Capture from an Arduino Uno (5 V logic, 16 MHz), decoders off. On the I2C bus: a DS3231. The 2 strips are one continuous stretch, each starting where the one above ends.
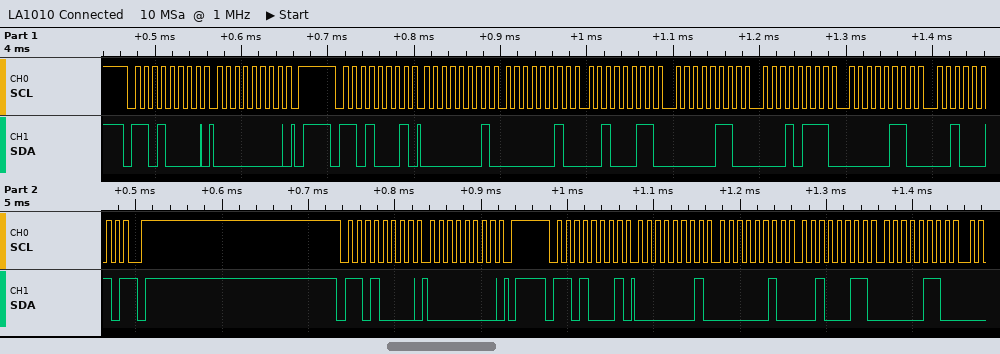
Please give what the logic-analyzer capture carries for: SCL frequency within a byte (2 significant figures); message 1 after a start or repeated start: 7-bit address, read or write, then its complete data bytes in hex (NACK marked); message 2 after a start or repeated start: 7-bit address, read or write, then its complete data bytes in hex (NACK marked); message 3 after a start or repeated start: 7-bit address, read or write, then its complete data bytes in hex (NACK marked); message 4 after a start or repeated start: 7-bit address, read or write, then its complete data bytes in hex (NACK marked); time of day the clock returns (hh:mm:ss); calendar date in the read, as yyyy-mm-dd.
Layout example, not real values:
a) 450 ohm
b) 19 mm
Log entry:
a) 100 kHz
b) 0x68 write: 00
c) 0x68 read: 01 02 23 06 17 06 22 NACK
d) 0x68 write: 00
e) 0x68 read: 01 02 23 06
f) 23:02:01
g) 2022-06-17
